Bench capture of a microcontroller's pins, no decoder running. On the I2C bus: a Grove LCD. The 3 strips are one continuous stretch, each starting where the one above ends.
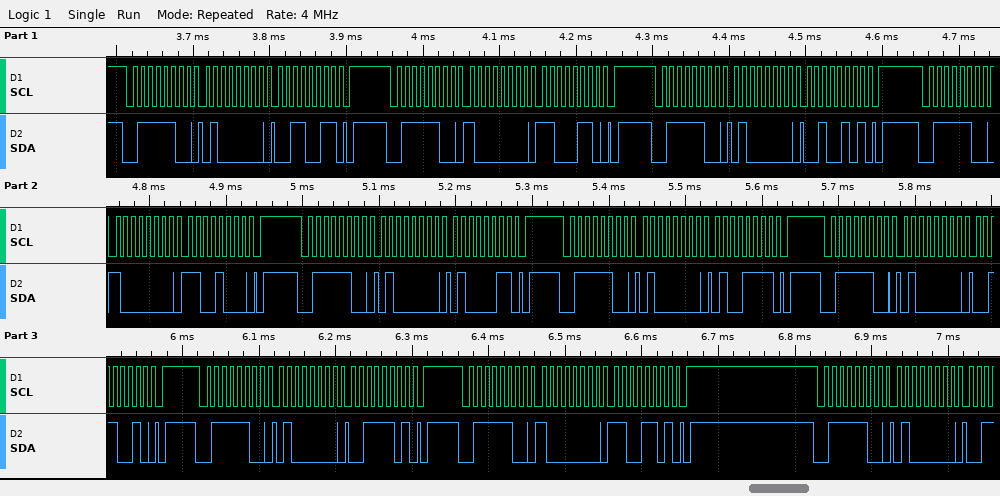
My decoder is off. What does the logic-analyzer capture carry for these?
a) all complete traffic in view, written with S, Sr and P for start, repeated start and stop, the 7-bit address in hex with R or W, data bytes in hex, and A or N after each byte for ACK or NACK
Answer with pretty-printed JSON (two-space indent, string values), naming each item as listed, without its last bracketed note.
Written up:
{
  "all complete traffic in view, written with S, Sr and P for start, repeated start and stop, the 7-bit address in hex with R or W, data bytes in hex, and A or N after each byte for ACK or NACK": "S 3EW A 40 A 33 A P S 3EW A 80 A C6 A P S 3EW A 40 A 25 A P S 3EW A 80 A C8 A P S 3EW A 40 A 43 A P S 3EW A 40 A 4F A P S 3EW A 40 A 32 A P S 3EW A 40 A 3D A P S 3EW A 80 A CD A P S 3EW A 40 A"
}
